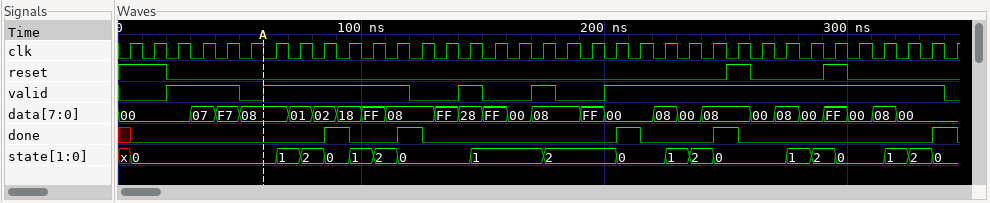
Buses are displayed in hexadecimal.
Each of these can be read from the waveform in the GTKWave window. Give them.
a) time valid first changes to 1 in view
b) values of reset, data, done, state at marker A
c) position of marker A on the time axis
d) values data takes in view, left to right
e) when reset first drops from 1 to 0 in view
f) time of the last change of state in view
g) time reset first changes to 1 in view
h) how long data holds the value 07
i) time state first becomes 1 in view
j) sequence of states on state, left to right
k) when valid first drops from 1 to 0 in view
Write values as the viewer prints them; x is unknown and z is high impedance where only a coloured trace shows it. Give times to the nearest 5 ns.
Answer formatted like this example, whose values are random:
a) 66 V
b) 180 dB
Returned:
a) 20 ns
b) reset=0, data=08, done=0, state=0
c) 60 ns
d) 00, 07, F7, 08, 01, 02, 18, FF, 08, FF, 28, FF, 00, 08, FF, 00, 08, 00, 08, 00, 08, 00, FF, 00, 08, 00
e) 20 ns
f) 335 ns
g) 250 ns
h) 10 ns
i) 65 ns
j) x, 0, 1, 2, 0, 1, 2, 0, 1, 2, 0, 1, 2, 0, 1, 2, 0, 1, 2, 0
k) 50 ns
